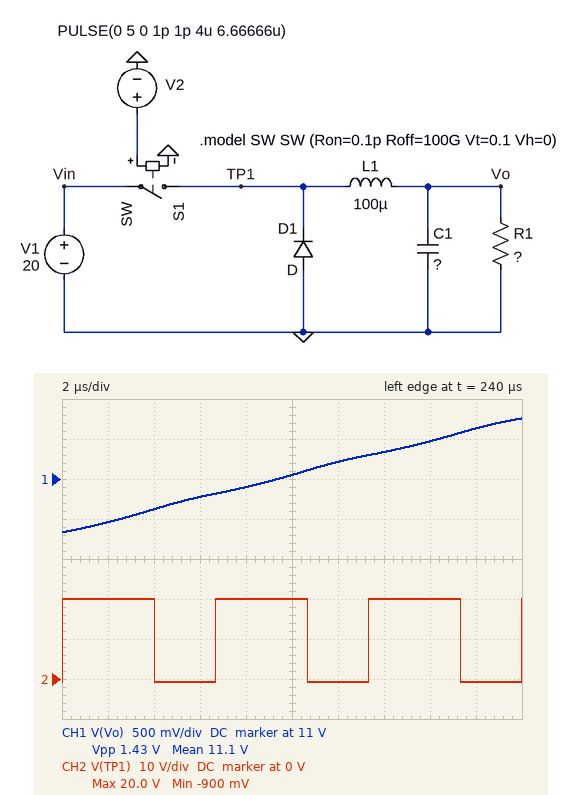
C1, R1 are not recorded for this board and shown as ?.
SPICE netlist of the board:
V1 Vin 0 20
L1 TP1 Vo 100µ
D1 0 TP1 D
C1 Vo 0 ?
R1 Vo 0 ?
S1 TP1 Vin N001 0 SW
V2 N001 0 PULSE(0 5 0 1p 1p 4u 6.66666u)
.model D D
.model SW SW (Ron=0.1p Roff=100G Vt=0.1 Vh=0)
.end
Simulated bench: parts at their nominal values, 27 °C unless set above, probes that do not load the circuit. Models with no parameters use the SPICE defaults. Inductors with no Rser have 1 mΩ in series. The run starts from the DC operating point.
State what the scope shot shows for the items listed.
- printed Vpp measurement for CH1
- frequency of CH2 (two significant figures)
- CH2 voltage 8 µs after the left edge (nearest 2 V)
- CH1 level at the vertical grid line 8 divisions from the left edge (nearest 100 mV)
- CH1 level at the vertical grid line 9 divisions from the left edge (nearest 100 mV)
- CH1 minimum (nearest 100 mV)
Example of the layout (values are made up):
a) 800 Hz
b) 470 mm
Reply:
a) 1.43 V
b) 150 kHz
c) 20 V
d) 11.5 V
e) 11.6 V
f) 10.3 V
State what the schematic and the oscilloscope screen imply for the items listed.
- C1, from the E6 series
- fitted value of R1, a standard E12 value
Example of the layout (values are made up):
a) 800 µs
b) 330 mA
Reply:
a) 10 µF
b) 8.2 Ω
